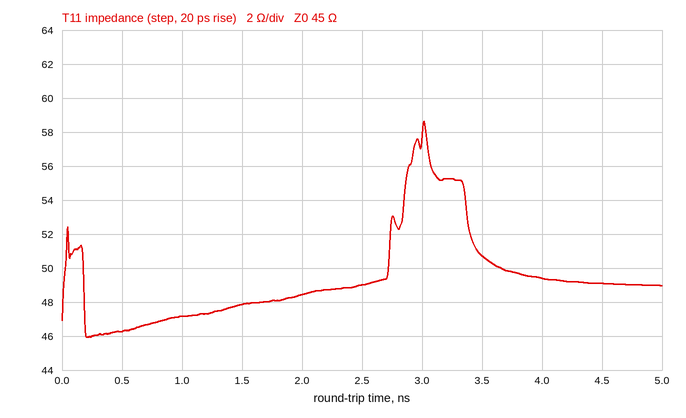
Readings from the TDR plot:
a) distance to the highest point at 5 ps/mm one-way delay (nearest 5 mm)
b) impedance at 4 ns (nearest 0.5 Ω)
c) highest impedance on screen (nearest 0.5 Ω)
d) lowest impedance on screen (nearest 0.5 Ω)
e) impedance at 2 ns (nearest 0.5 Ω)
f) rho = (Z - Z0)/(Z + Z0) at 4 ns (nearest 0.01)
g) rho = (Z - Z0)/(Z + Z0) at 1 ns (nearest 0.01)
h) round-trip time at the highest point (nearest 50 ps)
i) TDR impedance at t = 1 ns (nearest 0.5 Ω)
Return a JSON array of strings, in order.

["300 mm", "49.5 Ω", "58.5 Ω", "46.0 Ω", "48.5 Ω", "+0.05", "+0.02", "3.00 ns", "47.0 Ω"]
